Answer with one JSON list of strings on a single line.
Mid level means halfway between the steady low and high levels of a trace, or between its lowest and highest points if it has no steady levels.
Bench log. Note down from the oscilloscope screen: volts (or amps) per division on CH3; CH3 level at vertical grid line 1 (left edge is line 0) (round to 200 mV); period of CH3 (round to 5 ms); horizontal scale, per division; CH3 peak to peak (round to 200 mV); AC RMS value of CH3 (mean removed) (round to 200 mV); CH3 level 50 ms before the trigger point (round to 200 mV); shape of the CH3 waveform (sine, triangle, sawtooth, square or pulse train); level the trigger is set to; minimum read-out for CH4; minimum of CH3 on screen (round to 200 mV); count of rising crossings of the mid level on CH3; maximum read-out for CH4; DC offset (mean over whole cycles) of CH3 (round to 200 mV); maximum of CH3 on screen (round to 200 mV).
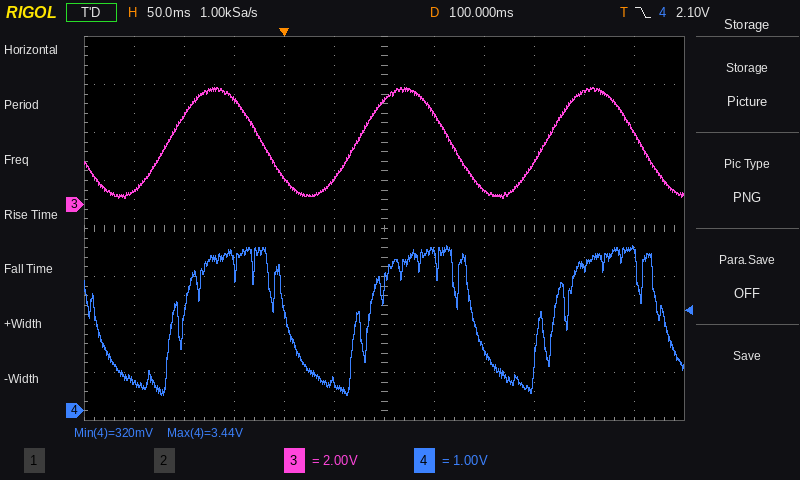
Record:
["2 V", "600 mV", "190 ms", "50 ms", "4.6 V", "1.6 V", "4.4 V", "sine", "2.10 V", "320 mV", "200 mV", "3", "3.44 V", "2.6 V", "4.8 V"]
